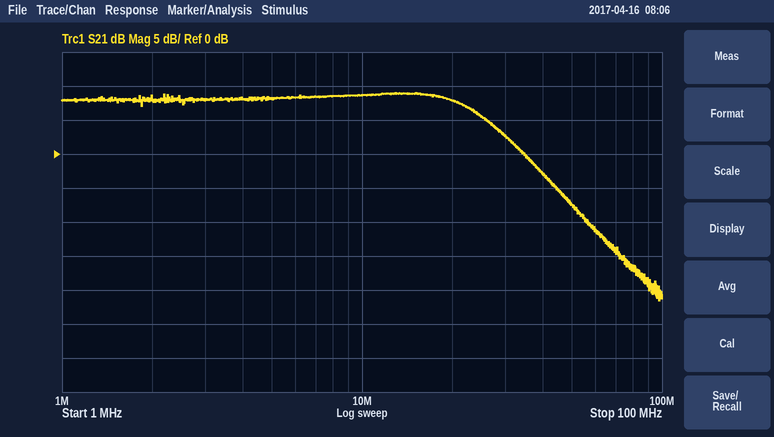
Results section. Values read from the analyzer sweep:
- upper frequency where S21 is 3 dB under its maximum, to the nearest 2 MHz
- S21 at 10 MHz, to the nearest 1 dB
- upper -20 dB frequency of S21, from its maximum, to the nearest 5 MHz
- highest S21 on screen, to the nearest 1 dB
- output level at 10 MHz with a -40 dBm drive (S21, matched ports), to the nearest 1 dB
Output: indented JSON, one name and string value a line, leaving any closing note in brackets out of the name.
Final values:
{
  "upper frequency where S21 is 3 dB under its maximum, to the nearest 2 MHz": "24 MHz",
  "S21 at 10 MHz, to the nearest 1 dB": "9 dB",
  "upper -20 dB frequency of S21, from its maximum, to the nearest 5 MHz": "60 MHz",
  "highest S21 on screen, to the nearest 1 dB": "9 dB",
  "output level at 10 MHz with a -40 dBm drive (S21, matched ports), to the nearest 1 dB": "-31 dBm"
}
